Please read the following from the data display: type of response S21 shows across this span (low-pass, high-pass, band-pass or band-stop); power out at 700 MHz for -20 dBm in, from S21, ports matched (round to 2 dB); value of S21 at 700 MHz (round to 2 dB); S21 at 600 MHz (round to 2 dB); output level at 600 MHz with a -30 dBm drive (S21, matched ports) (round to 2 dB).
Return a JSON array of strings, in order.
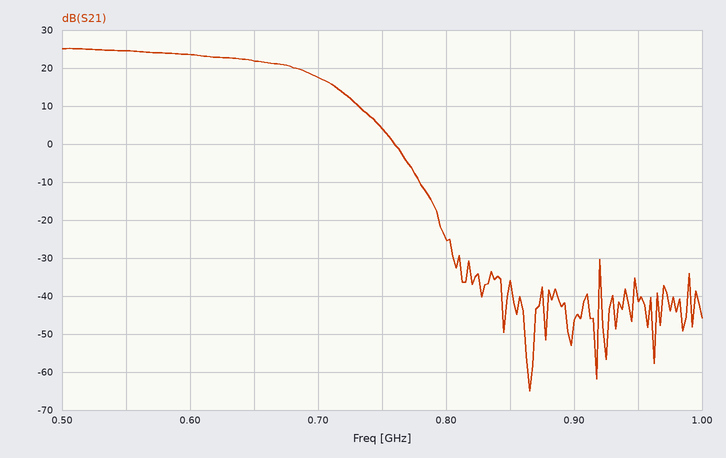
["low-pass", "-2 dBm", "18 dB", "24 dB", "-6 dBm"]
